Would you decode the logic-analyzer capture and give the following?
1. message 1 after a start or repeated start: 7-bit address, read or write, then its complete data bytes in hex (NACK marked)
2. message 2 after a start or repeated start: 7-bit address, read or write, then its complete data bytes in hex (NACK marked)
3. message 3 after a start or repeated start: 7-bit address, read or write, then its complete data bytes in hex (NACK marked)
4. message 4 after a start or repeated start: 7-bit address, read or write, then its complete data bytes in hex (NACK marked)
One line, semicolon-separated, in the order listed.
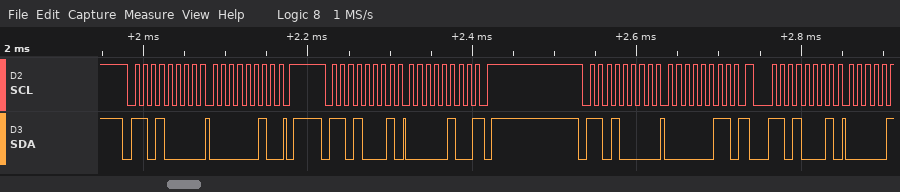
0x68 write: 02; 0x68 read: 04 NACK; 0x68 write: 03; 0x68 read
